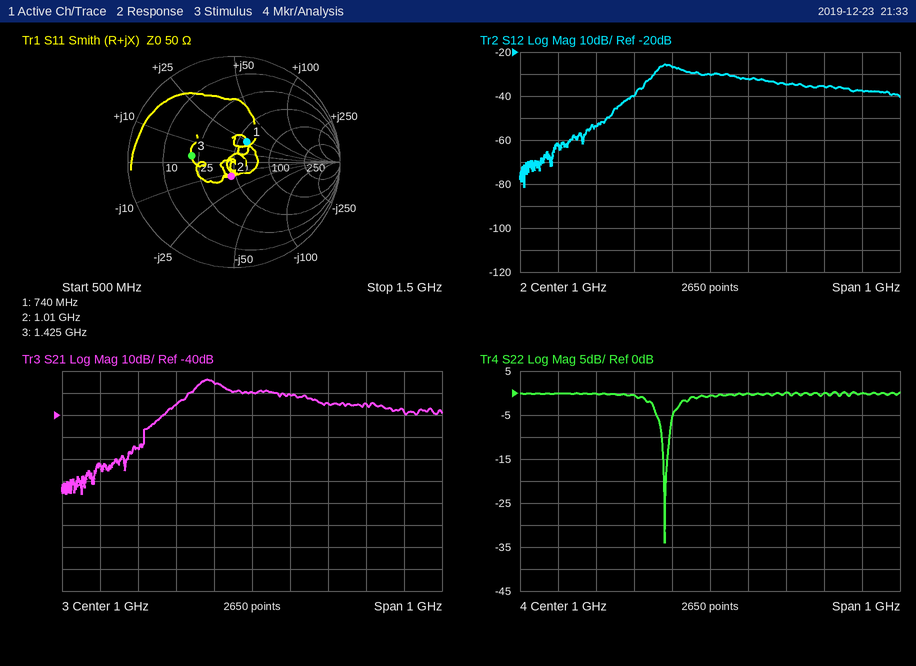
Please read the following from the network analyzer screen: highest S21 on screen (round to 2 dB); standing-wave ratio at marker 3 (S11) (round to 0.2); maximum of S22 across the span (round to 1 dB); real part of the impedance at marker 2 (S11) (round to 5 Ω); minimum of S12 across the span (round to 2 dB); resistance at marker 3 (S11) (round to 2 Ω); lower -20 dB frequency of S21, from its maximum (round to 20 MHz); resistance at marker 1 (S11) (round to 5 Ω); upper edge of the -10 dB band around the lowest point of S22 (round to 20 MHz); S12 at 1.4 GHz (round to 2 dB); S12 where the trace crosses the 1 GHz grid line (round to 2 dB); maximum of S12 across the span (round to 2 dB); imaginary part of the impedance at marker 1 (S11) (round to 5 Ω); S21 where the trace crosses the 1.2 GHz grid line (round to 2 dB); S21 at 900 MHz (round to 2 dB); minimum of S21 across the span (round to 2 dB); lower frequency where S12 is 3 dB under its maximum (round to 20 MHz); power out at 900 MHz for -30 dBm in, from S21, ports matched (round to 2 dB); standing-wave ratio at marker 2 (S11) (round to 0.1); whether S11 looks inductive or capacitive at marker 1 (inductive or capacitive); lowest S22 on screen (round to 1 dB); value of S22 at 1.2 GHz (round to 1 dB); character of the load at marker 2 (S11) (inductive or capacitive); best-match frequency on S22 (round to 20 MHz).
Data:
-24 dB
2.4
0 dB
45 Ω
-82 dB
22 Ω
740 MHz
60 Ω
900 MHz
-38 dB
-30 dB
-26 dB
+25 Ω
-34 dB
-26 dB
-76 dB
860 MHz
-56 dBm
1.3
inductive
-34 dB
0 dB
capacitive
880 MHz
